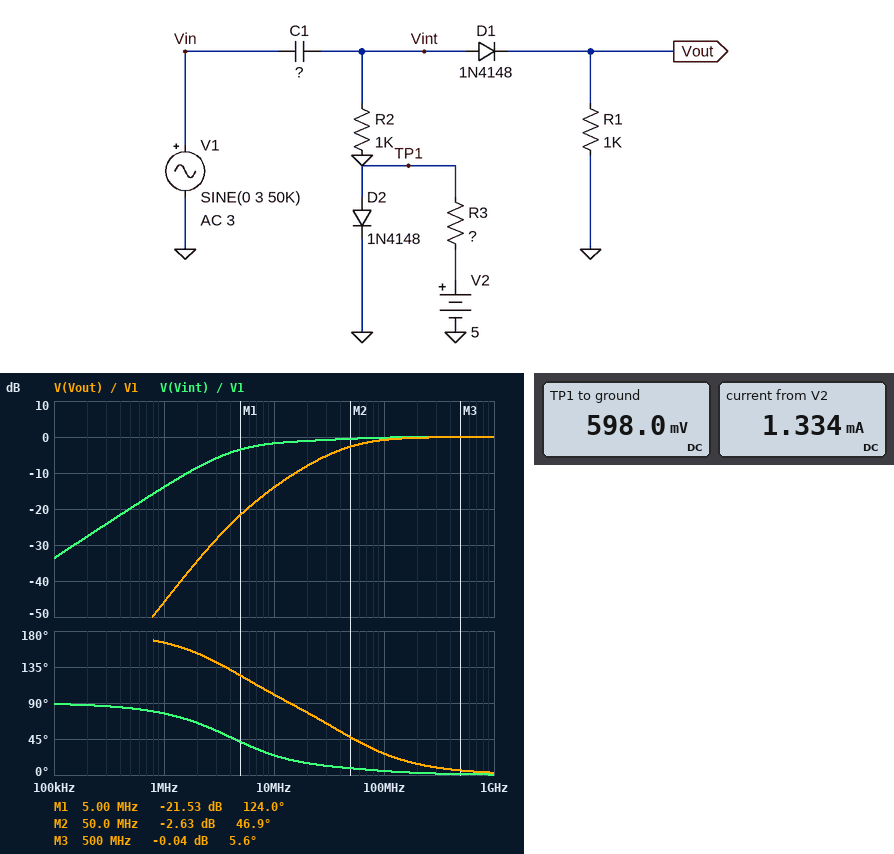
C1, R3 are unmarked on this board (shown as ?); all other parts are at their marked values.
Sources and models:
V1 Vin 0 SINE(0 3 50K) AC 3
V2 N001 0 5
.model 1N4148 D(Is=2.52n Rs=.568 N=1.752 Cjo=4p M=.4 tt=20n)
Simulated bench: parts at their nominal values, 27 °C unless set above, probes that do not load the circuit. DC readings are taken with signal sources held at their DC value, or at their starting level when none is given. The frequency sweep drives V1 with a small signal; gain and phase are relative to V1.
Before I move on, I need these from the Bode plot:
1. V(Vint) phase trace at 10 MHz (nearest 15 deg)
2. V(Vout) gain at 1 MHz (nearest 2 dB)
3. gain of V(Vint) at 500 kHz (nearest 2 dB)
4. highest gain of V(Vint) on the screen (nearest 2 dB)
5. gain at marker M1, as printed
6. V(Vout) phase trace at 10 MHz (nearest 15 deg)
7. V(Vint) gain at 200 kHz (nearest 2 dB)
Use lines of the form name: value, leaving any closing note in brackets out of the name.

V(Vint) phase trace at 10 MHz: 30 deg
V(Vout) gain at 1 MHz: -46 dB
gain of V(Vint) at 500 kHz: -20 dB
highest gain of V(Vint) on the screen: 0 dB
gain at marker M1, as printed: -21.53 dB
V(Vout) phase trace at 10 MHz: 105 deg
V(Vint) gain at 200 kHz: -28 dB
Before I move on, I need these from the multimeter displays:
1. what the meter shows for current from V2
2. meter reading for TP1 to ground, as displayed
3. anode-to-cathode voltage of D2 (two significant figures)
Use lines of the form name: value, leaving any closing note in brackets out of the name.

what the meter shows for current from V2: 1.334 mA
meter reading for TP1 to ground, as displayed: 598.0 mV
anode-to-cathode voltage of D2: 600 mV
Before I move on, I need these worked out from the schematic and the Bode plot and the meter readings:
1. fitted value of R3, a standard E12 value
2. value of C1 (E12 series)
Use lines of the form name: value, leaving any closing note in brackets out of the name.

fitted value of R3, a standard E12 value: 3.3 kΩ
value of C1: 33 pF
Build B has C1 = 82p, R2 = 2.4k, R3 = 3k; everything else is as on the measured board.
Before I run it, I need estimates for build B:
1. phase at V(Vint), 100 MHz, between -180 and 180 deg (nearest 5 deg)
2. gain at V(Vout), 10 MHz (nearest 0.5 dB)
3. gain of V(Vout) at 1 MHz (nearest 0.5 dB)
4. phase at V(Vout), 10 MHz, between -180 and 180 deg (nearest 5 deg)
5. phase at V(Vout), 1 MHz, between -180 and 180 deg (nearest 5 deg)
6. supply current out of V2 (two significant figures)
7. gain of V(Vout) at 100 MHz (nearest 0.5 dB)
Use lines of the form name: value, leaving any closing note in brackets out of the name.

phase at V(Vint), 100 MHz, between -180 and 180 deg: 0 deg
gain at V(Vout), 10 MHz: -12.5 dB
gain of V(Vout) at 1 MHz: -34.5 dB
phase at V(Vout), 10 MHz, between -180 and 180 deg: 80 deg
phase at V(Vout), 1 MHz, between -180 and 180 deg: 125 deg
supply current out of V2: 1.5 mA
gain of V(Vout) at 100 MHz: -0.5 dB
